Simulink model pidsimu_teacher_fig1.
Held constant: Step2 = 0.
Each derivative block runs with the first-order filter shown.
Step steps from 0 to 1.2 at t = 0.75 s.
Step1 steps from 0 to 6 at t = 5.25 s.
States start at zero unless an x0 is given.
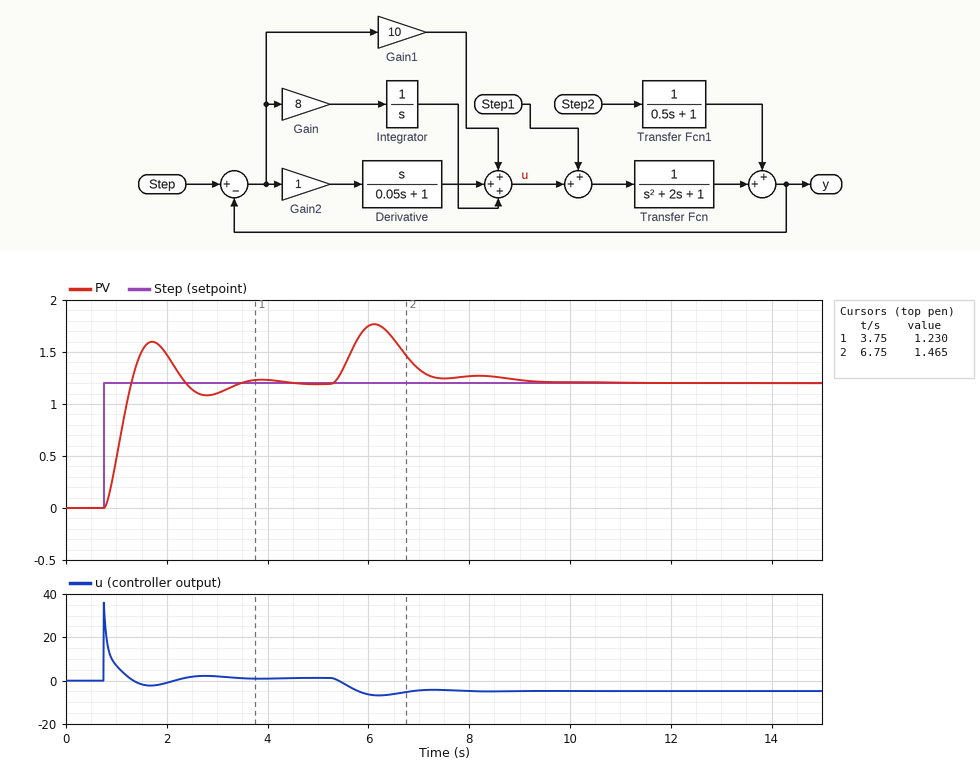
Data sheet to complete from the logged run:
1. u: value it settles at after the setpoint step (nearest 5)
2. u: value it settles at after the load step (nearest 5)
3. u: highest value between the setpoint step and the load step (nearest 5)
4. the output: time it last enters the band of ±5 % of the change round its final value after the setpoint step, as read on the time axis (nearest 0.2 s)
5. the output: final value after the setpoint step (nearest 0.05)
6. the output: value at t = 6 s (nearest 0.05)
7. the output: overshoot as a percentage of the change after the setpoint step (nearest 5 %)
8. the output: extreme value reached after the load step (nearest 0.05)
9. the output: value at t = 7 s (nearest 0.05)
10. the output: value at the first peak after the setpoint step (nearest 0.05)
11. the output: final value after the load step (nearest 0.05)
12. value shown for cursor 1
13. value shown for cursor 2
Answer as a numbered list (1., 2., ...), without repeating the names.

1. 0
2. -5
3. 35
4. 3.2 s
5. 1.20
6. 1.75
7. 35 %
8. 1.75
9. 1.35
10. 1.60
11. 1.20
12. 1.230
13. 1.465
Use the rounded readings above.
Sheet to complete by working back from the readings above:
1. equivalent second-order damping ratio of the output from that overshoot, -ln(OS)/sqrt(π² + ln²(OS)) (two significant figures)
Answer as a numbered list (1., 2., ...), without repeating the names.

1. 0.32
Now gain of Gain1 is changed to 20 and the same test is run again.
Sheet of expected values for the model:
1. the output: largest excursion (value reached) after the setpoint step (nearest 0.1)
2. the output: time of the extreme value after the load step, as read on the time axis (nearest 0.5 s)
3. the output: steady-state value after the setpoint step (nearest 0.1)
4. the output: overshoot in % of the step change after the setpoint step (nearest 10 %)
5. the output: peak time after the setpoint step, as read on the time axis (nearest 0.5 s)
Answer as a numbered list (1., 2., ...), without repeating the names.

1. 1.7
2. 6.0 s
3. 1.2
4. 40 %
5. 1.5 s
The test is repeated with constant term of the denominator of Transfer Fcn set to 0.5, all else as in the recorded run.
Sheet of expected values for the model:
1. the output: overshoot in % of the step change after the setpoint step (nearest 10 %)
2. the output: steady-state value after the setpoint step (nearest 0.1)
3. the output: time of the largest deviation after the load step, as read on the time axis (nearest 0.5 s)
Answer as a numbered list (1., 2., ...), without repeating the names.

1. 40 %
2. 1.2
3. 6.0 s
